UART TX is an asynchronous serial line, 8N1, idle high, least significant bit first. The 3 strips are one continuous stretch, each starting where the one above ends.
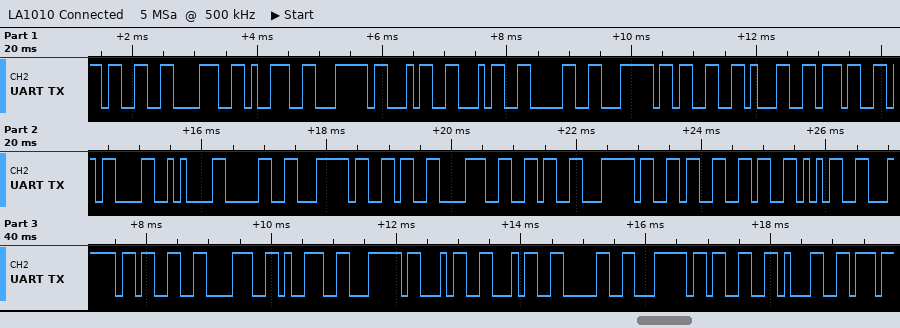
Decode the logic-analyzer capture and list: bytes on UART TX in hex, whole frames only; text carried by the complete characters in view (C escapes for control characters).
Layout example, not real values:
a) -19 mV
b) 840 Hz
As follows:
a) 0x33 0x38 0x39 0x7C 0x34 0x34 0x30 0x7C 0x33 0x31 0x37 0x0D 0x0A 0x30 0x7C 0x36 0x38 0x36 0x7C 0x36 0x36 0x35 0x7C 0x33 0x38 0x39 0x7C 0x34 0x34 0x30 0x7C 0x33 0x31
b) "389|440|317\r\n0|686|665|389|440|31"
